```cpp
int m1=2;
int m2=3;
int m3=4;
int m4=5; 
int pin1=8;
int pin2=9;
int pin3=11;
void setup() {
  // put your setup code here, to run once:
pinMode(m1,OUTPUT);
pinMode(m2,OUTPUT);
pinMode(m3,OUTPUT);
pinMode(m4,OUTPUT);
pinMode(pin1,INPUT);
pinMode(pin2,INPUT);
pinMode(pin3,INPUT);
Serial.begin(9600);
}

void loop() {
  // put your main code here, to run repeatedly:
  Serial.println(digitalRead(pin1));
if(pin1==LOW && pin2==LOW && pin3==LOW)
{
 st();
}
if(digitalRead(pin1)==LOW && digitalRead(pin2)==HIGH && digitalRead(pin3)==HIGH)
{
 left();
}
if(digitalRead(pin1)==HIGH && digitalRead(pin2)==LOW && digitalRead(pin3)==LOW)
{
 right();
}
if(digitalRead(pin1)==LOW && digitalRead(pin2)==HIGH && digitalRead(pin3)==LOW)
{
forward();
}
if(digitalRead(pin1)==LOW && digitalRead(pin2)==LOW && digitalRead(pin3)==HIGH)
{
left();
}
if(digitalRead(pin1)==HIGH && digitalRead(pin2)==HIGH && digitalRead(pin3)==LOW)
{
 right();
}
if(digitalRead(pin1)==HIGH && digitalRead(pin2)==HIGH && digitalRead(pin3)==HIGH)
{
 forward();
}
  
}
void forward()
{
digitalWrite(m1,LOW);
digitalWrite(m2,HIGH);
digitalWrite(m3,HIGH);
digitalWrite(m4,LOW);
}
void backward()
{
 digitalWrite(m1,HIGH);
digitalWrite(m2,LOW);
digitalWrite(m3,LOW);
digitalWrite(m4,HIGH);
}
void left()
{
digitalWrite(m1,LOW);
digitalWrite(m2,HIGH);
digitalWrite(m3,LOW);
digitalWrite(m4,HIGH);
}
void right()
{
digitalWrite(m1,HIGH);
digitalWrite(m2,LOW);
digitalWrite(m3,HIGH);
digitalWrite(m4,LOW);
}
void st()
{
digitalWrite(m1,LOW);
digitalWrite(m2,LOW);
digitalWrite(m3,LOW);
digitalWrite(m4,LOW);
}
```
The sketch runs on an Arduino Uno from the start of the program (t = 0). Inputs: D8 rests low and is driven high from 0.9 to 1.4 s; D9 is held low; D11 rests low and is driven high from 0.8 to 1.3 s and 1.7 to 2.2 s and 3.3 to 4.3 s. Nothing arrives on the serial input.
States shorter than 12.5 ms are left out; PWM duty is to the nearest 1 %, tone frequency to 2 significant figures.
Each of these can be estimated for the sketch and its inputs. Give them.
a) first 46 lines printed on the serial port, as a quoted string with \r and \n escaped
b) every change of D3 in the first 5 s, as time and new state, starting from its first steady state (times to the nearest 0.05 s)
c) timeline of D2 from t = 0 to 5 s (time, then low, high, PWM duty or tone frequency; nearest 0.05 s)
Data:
"0\r\n0\r\n0\r\n0\r\n0\r\n0\r\n0\r\n0\r\n0\r\n0\r\n0\r\n0\r\n0\r\n0\r\n0\r\n0\r\n0\r\n0\r\n0\r\n0\r\n0\r\n0\r\n0\r\n0\r\n0\r\n0\r\n0\r\n0\r\n0\r\n0\r\n0\r\n0\r\n0\r\n0\r\n0\r\n0\r\n0\r\n0\r\n0\r\n0\r\n0\r\n0\r\n0\r\n0\r\n0\r\n0\r\n"
0 s low; 0.8 s high; 1.3 s low; 1.7 s high
0 s low; 1.3 s high; 1.7 s low
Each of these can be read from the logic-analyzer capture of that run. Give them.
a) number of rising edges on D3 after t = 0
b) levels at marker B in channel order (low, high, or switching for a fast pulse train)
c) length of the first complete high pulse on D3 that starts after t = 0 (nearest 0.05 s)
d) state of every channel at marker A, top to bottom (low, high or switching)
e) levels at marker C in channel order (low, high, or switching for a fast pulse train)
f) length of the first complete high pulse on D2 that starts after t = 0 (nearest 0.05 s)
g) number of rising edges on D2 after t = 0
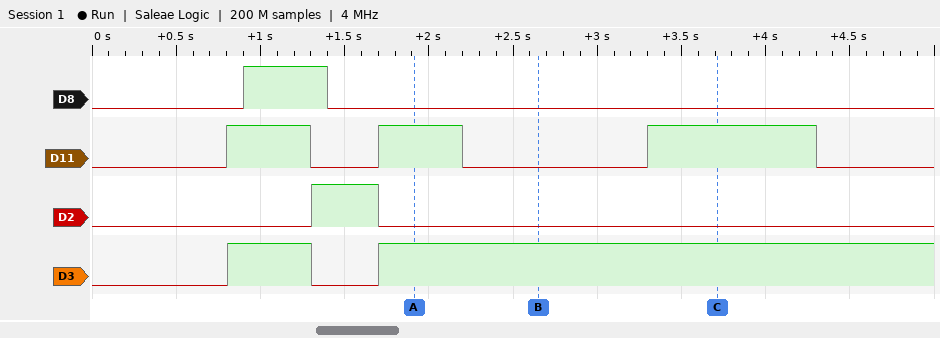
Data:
2
D8 low, D11 low, D2 low, D3 high
0.50 s
D8 low, D11 high, D2 low, D3 high
D8 low, D11 high, D2 low, D3 high
0.40 s
1
